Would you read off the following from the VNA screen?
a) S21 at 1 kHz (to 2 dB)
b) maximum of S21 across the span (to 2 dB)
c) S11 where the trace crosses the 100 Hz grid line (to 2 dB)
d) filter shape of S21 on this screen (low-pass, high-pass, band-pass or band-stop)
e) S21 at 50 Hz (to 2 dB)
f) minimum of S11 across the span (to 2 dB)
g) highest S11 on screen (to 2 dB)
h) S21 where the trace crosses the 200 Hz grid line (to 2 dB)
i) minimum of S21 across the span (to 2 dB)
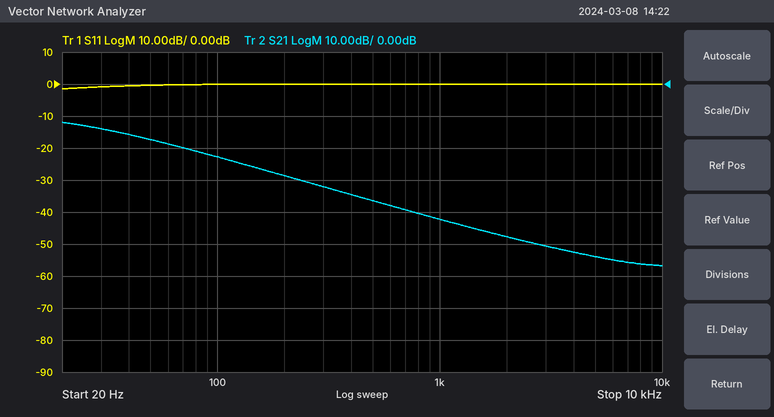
-42 dB
-12 dB
0 dB
low-pass
-18 dB
-2 dB
0 dB
-28 dB
-56 dB
